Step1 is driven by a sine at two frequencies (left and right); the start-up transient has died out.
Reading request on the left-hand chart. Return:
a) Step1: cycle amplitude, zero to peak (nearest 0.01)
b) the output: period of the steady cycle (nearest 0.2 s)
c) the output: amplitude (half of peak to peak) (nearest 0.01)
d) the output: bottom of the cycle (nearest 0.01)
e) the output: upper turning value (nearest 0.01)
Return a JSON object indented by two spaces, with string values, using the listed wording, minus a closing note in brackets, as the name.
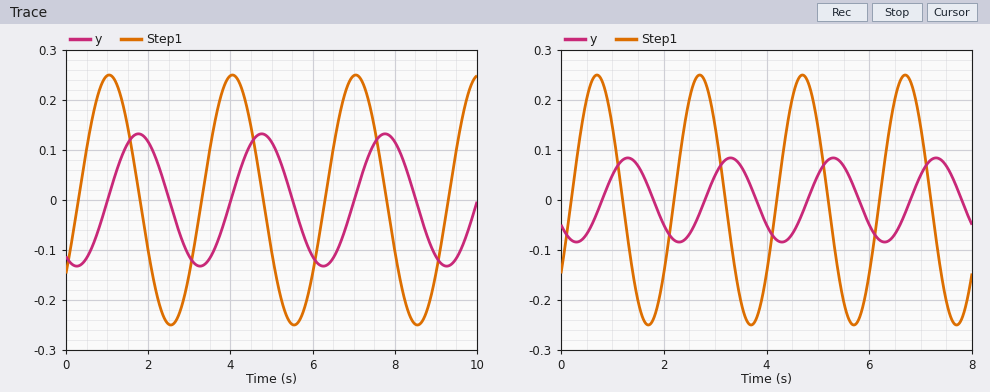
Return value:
{
  "Step1: cycle amplitude, zero to peak": "0.25",
  "the output: period of the steady cycle": "3.0 s",
  "the output: amplitude (half of peak to peak)": "0.13",
  "the output: bottom of the cycle": "-0.13",
  "the output: upper turning value": "0.13"
}
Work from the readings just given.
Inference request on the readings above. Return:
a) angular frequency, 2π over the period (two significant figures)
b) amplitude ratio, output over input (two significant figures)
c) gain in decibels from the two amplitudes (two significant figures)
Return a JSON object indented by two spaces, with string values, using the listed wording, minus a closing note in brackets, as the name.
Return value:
{
  "angular frequency, 2π over the period": "2.1 rad/s",
  "amplitude ratio, output over input": "0.52",
  "gain in decibels from the two amplitudes": "-5.7 dB"
}
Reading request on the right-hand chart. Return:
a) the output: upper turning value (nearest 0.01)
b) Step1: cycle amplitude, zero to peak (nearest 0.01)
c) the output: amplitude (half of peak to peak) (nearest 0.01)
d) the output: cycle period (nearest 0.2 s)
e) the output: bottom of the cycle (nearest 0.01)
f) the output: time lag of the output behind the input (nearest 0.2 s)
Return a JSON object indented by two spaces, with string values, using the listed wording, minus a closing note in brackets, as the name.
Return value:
{
  "the output: upper turning value": "0.08",
  "Step1: cycle amplitude, zero to peak": "0.25",
  "the output: amplitude (half of peak to peak)": "0.08",
  "the output: cycle period": "2.0 s",
  "the output: bottom of the cycle": "-0.08",
  "the output: time lag of the output behind the input": "0.6 s"
}
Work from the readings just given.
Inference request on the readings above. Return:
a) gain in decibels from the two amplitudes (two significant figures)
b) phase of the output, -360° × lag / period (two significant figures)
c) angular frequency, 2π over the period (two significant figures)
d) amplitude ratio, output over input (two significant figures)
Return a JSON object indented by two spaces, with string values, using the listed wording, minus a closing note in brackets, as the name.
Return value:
{
  "gain in decibels from the two amplitudes": "-9.9 dB",
  "phase of the output, -360° × lag / period": "-110°",
  "angular frequency, 2π over the period": "3.1 rad/s",
  "amplitude ratio, output over input": "0.32"
}
